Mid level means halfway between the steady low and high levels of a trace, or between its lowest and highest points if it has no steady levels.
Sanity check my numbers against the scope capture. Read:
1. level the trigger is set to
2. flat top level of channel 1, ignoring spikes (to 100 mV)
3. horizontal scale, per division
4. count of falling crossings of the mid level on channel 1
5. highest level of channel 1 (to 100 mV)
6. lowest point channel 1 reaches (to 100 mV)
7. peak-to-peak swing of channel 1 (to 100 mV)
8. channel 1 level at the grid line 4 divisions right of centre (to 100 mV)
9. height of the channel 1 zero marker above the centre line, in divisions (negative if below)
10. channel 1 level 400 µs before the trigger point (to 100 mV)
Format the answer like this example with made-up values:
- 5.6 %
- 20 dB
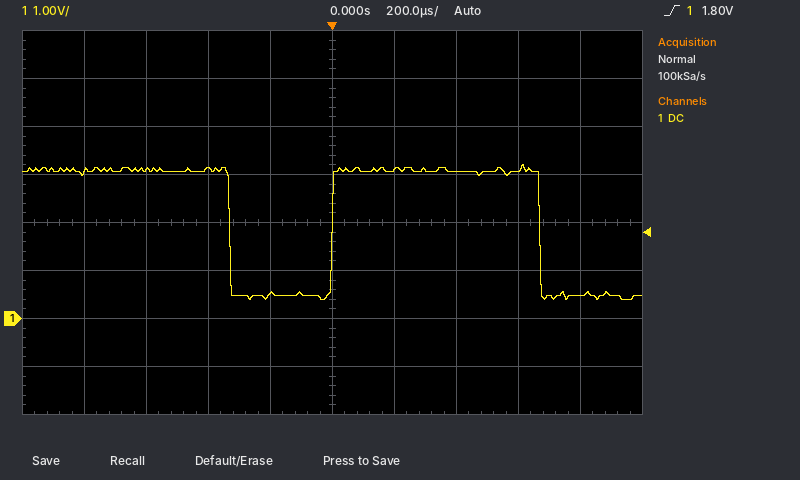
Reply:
- 1.80 V
- 3.1 V
- 200 µs
- 2
- 3.2 V
- 400 mV
- 2.8 V
- 500 mV
- -2.0 div
- 3.1 V
